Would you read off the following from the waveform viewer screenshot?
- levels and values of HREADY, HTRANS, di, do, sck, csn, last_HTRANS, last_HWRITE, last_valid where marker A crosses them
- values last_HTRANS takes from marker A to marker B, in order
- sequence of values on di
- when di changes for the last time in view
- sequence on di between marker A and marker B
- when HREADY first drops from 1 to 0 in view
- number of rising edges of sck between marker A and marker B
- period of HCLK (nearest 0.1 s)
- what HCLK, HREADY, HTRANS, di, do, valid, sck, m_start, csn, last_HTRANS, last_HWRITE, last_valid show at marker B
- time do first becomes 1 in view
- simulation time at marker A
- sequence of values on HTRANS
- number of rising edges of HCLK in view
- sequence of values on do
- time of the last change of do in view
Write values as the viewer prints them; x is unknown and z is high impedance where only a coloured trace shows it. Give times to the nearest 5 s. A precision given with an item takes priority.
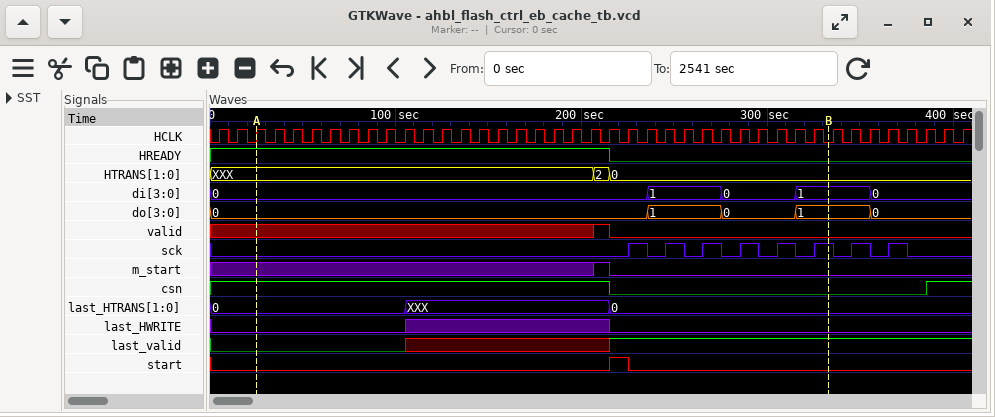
HREADY=1, HTRANS=XXX, di=0, do=0, sck=0, csn=1, last_HTRANS=0, last_HWRITE=0, last_valid=0
0, XXX, 0
0, 1, 0, 1, 0
355 s
0, 1, 0, 1
215 s
6
10 s
HCLK=0, HREADY=0, HTRANS=0, di=1, do=1, valid=0, sck=1, m_start=0, csn=0, last_HTRANS=0, last_HWRITE=0, last_valid=1
235 s
25 s
XXX, 2, 0
41
0, 1, 0, 1, 0
355 s
